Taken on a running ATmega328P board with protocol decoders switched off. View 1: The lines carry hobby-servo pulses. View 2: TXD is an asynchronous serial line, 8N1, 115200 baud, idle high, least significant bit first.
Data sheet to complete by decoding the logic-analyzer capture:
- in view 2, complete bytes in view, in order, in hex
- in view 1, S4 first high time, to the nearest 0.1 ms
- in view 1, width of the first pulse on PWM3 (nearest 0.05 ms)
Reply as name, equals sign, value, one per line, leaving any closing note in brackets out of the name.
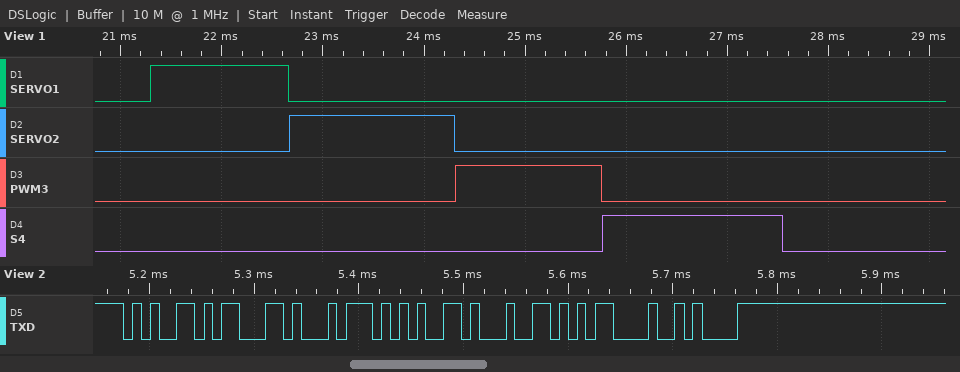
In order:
in view 2, complete bytes in view, in order, in hex = 65 63 74 65 64 0D 0A
in view 1, S4 first high time, to the nearest 0.1 ms = 1.8 ms
in view 1, width of the first pulse on PWM3 = 1.45 ms
